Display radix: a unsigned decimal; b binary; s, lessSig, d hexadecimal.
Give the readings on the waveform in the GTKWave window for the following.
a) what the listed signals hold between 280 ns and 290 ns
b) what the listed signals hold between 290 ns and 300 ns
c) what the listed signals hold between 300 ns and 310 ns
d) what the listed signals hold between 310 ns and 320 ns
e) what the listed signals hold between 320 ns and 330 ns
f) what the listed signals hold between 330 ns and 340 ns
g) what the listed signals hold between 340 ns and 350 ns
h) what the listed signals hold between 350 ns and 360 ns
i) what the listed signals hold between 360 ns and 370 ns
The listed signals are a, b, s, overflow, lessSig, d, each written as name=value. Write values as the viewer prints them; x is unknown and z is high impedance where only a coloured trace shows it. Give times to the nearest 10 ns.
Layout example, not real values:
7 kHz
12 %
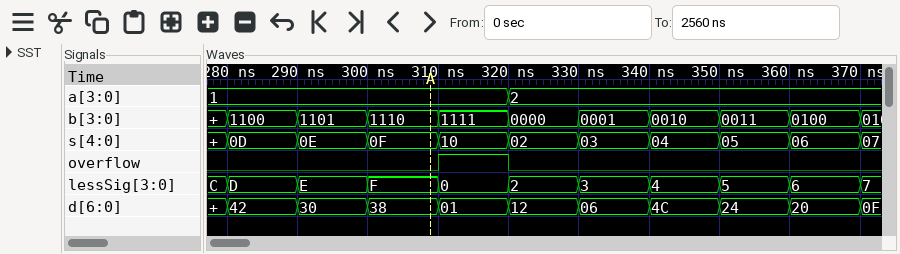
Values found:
a=1, b=1100, s=0D, overflow=0, lessSig=D, d=42
a=1, b=1101, s=0E, overflow=0, lessSig=E, d=30
a=1, b=1110, s=0F, overflow=0, lessSig=F, d=38
a=1, b=1111, s=10, overflow=1, lessSig=0, d=01
a=2, b=0000, s=02, overflow=0, lessSig=2, d=12
a=2, b=0001, s=03, overflow=0, lessSig=3, d=06
a=2, b=0010, s=04, overflow=0, lessSig=4, d=4C
a=2, b=0011, s=05, overflow=0, lessSig=5, d=24
a=2, b=0100, s=06, overflow=0, lessSig=6, d=20
